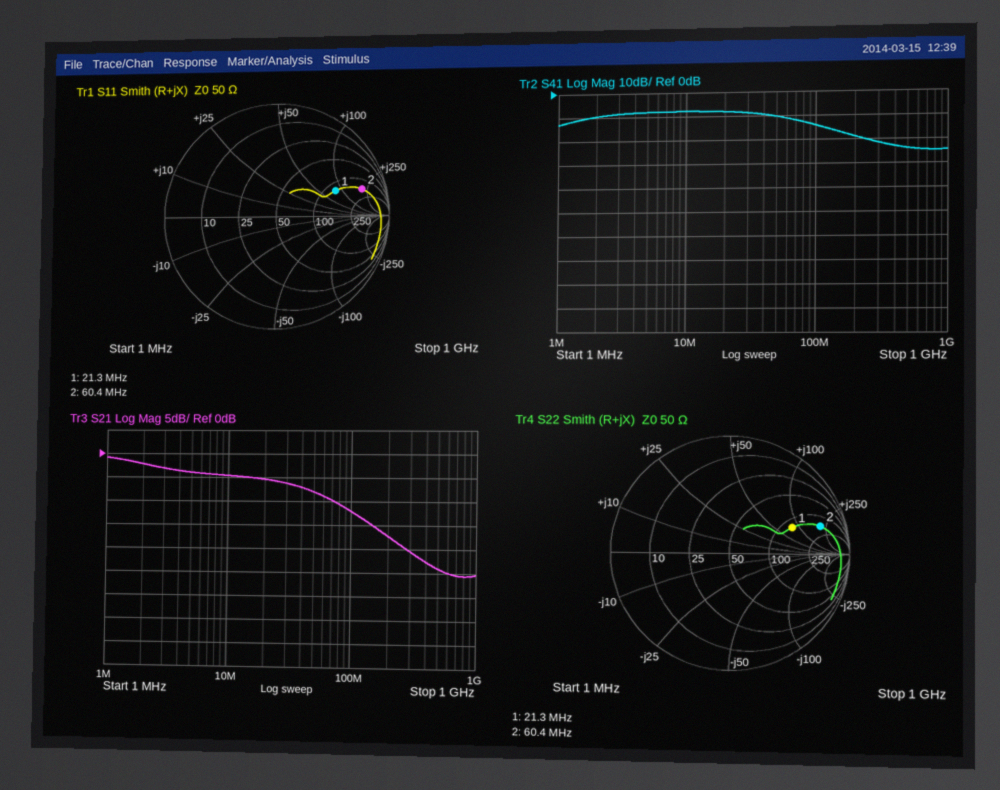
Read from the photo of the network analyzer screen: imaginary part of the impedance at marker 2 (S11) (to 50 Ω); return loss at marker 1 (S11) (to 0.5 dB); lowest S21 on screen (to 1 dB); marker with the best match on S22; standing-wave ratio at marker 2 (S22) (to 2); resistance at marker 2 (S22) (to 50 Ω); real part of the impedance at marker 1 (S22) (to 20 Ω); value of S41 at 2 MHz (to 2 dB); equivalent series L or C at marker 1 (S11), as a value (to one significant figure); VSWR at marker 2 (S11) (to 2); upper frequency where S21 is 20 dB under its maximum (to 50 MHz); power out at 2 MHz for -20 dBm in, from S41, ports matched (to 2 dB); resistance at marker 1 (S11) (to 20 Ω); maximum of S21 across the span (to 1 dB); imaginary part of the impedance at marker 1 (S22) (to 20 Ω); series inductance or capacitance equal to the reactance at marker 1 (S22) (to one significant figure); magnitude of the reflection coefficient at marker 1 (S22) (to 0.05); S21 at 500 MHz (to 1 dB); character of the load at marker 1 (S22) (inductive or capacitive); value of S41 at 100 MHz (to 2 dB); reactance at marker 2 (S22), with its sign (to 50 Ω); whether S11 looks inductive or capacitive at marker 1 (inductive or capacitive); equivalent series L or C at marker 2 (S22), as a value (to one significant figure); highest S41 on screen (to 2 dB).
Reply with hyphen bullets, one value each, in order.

- +200 Ω
- 5.0 dB
- -26 dB
- marker 1
- 8
- 150 Ω
- 120 Ω
- -10 dB
- 600 nH
- 8
- 300 MHz
- -30 dBm
- 120 Ω
- -1 dB
- +80 Ω
- 600 nH
- 0.55
- -24 dB
- inductive
- -14 dB
- +200 Ω
- inductive
- 500 nH
- -8 dB
